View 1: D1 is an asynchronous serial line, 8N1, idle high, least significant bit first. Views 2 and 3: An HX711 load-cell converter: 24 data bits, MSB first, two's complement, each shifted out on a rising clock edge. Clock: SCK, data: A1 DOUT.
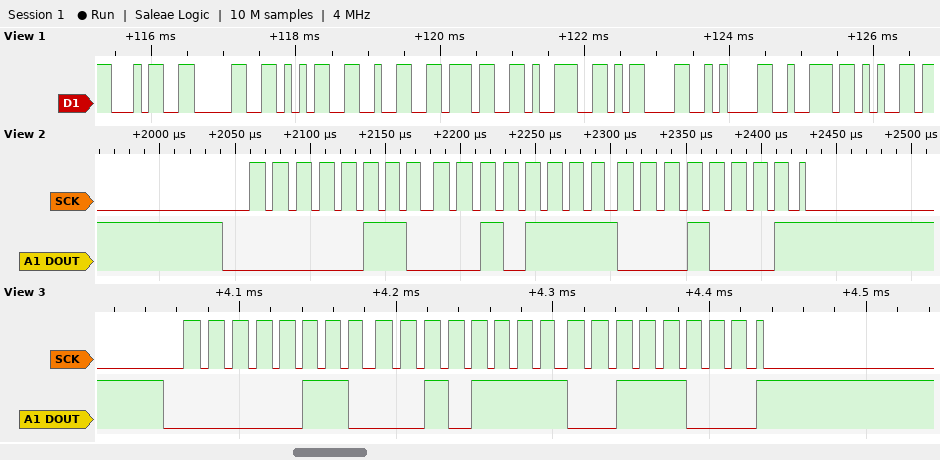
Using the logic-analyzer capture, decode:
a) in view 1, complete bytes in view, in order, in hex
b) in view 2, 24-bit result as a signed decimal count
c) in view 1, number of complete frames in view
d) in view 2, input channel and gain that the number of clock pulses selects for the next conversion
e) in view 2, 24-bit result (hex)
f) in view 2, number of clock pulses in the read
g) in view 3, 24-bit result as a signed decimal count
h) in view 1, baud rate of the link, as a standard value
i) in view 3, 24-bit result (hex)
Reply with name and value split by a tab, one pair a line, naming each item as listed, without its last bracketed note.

in view 1, complete bytes in view, in order, in hex	34 30 35 32 37 39 0D 0A 72 65
in view 2, 24-bit result as a signed decimal count	405265
in view 1, number of complete frames in view	10
in view 2, input channel and gain that the number of clock pulses selects for the next conversion	channel A, gain 128
in view 2, 24-bit result	0x062F11
in view 2, number of clock pulses in the read	25
in view 3, 24-bit result as a signed decimal count	405304
in view 1, baud rate of the link, as a standard value	9600 baud
in view 3, 24-bit result	0x062F38
